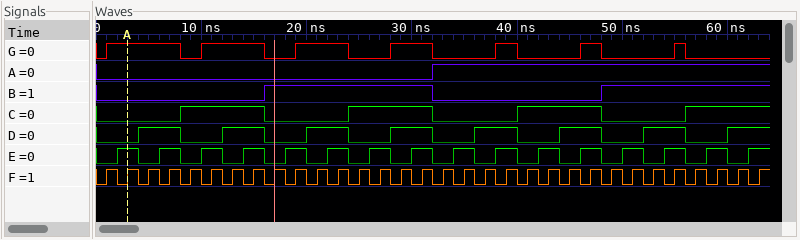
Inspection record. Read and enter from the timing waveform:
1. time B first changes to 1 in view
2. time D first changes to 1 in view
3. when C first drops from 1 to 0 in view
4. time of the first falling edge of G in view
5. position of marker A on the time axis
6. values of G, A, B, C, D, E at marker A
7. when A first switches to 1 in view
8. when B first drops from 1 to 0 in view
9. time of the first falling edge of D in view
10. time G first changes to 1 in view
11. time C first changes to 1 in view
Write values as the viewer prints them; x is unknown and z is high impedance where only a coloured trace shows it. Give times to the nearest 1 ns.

16 ns
4 ns
16 ns
8 ns
3 ns
G=1, A=0, B=0, C=0, D=0, E=1
32 ns
32 ns
8 ns
1 ns
8 ns
